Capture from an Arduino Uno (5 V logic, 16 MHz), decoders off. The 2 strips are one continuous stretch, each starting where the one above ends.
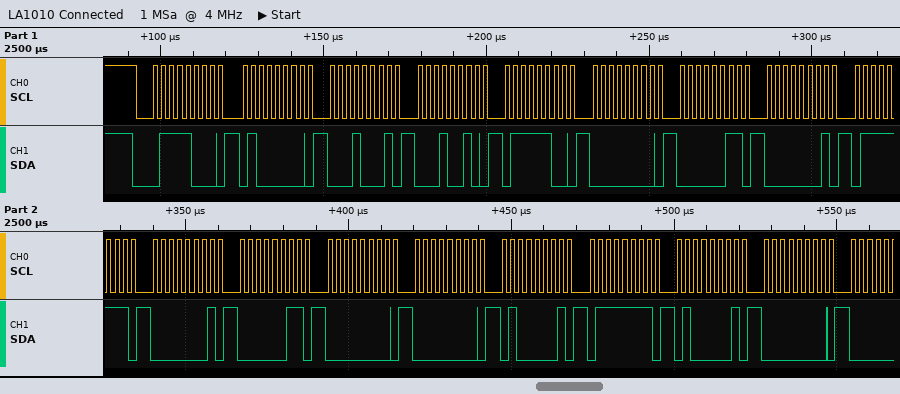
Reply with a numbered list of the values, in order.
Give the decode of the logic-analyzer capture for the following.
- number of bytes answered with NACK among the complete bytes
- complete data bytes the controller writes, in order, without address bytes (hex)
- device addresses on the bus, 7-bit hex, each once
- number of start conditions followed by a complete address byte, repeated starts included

1. 0
2. 40 11 12 7C 00 03 01 7F 01 03 00 00 41 7F 41 00
3. 0x3C
4. 1
